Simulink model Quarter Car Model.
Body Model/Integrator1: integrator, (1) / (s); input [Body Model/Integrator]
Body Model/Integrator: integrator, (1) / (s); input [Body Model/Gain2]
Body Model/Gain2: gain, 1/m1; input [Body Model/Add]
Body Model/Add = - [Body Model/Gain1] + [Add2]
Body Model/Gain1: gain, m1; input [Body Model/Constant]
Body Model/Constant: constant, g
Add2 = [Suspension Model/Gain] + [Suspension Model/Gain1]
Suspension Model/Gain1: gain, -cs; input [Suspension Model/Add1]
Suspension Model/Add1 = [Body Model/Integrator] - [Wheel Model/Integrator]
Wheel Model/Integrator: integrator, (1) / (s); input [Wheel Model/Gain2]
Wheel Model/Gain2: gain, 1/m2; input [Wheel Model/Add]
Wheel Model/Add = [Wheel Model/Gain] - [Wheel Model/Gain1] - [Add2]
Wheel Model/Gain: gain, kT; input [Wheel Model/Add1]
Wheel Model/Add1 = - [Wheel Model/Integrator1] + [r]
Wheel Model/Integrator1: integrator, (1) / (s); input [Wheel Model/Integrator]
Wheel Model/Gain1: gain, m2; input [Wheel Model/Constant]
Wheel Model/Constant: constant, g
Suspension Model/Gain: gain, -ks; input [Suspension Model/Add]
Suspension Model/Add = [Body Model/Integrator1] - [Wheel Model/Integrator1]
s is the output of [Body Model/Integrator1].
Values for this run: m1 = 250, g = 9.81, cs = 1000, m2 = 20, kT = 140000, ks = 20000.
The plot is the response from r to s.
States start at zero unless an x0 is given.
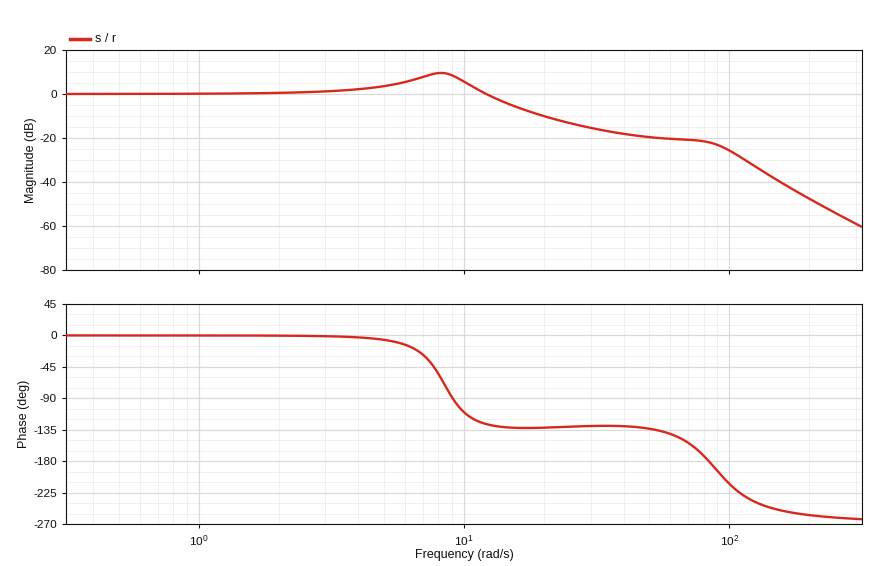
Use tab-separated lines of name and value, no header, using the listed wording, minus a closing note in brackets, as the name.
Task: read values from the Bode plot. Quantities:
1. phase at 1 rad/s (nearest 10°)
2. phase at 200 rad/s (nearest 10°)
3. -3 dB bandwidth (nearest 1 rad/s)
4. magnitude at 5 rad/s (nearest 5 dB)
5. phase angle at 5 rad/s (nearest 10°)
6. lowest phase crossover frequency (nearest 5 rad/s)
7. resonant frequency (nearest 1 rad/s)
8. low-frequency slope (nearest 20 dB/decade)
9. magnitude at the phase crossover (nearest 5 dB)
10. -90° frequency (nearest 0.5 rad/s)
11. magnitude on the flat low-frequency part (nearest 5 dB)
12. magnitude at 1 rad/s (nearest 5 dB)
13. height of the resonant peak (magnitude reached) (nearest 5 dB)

phase at 1 rad/s	0°
phase at 200 rad/s	-260°
-3 dB bandwidth	14 rad/s
magnitude at 5 rad/s	5 dB
phase angle at 5 rad/s	-10°
lowest phase crossover frequency	85 rad/s
resonant frequency	8 rad/s
low-frequency slope	0 dB/decade
magnitude at the phase crossover	-20 dB
-90° frequency	9.0 rad/s
magnitude on the flat low-frequency part	0 dB
magnitude at 1 rad/s	0 dB
height of the resonant peak (magnitude reached)	10 dB
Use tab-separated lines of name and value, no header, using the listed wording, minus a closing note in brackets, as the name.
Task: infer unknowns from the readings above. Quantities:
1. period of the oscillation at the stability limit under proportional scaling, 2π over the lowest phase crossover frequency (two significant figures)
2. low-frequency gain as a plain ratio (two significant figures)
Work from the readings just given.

period of the oscillation at the stability limit under proportional scaling, 2π over the lowest phase crossover frequency	0.074 s
low-frequency gain as a plain ratio	1.0
